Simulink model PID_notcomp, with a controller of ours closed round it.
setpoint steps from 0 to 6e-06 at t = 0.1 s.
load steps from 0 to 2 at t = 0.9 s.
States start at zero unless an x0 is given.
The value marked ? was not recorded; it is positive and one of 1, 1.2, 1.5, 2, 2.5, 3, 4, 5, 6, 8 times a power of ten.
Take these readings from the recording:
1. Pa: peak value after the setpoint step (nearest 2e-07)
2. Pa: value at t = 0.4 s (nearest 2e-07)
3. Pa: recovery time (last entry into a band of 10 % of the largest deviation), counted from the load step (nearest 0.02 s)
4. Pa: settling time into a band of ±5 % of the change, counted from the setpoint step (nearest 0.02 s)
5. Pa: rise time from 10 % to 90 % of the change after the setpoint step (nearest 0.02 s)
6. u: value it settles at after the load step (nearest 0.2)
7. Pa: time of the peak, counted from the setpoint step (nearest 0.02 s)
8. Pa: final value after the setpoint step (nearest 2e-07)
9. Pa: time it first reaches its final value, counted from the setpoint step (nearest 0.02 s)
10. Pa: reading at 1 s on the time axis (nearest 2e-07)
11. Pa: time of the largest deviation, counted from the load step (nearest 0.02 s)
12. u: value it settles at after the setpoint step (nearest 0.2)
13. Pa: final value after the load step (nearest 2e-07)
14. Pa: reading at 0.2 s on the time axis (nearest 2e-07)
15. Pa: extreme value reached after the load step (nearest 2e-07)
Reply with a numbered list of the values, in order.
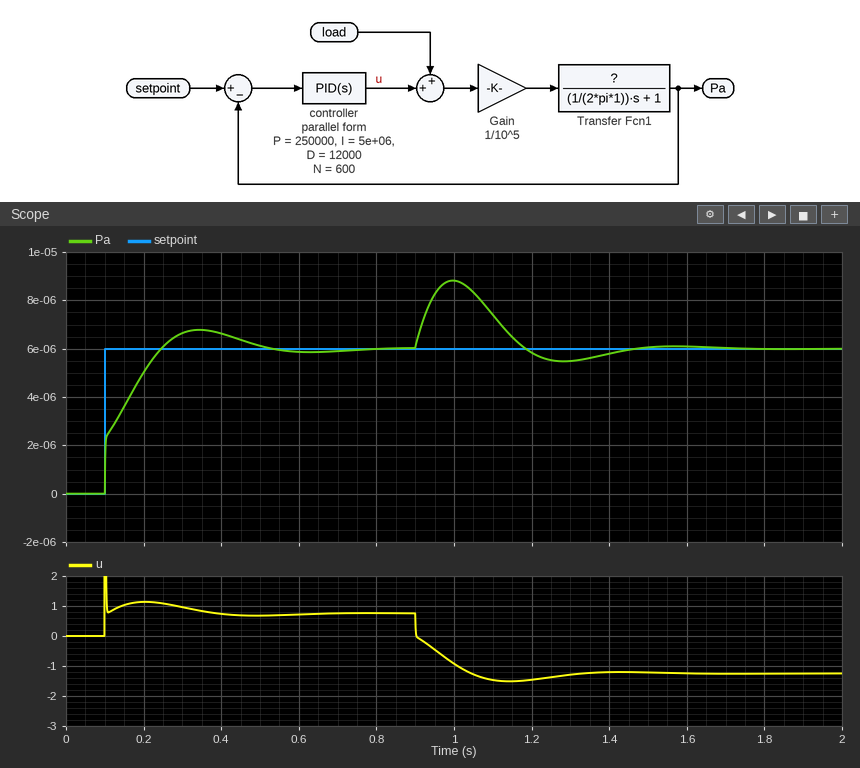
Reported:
1. 0.0000068
2. 0.0000066
3. 0.48 s
4. 0.36 s
5. 0.12 s
6. -1.2
7. 0.24 s
8. 0.0000060
9. 0.14 s
10. 0.0000088
11. 0.10 s
12. 0.8
13. 0.0000060
14. 0.0000050
15. 0.0000088
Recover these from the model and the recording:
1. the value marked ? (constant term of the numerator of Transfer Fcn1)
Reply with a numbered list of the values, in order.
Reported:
1. 0.8
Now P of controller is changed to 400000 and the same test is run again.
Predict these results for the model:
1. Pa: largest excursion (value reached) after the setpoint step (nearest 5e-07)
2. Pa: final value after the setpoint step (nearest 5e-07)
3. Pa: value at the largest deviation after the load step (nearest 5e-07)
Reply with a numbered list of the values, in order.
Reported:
1. 0.0000065
2. 0.0000060
3. 0.0000085
